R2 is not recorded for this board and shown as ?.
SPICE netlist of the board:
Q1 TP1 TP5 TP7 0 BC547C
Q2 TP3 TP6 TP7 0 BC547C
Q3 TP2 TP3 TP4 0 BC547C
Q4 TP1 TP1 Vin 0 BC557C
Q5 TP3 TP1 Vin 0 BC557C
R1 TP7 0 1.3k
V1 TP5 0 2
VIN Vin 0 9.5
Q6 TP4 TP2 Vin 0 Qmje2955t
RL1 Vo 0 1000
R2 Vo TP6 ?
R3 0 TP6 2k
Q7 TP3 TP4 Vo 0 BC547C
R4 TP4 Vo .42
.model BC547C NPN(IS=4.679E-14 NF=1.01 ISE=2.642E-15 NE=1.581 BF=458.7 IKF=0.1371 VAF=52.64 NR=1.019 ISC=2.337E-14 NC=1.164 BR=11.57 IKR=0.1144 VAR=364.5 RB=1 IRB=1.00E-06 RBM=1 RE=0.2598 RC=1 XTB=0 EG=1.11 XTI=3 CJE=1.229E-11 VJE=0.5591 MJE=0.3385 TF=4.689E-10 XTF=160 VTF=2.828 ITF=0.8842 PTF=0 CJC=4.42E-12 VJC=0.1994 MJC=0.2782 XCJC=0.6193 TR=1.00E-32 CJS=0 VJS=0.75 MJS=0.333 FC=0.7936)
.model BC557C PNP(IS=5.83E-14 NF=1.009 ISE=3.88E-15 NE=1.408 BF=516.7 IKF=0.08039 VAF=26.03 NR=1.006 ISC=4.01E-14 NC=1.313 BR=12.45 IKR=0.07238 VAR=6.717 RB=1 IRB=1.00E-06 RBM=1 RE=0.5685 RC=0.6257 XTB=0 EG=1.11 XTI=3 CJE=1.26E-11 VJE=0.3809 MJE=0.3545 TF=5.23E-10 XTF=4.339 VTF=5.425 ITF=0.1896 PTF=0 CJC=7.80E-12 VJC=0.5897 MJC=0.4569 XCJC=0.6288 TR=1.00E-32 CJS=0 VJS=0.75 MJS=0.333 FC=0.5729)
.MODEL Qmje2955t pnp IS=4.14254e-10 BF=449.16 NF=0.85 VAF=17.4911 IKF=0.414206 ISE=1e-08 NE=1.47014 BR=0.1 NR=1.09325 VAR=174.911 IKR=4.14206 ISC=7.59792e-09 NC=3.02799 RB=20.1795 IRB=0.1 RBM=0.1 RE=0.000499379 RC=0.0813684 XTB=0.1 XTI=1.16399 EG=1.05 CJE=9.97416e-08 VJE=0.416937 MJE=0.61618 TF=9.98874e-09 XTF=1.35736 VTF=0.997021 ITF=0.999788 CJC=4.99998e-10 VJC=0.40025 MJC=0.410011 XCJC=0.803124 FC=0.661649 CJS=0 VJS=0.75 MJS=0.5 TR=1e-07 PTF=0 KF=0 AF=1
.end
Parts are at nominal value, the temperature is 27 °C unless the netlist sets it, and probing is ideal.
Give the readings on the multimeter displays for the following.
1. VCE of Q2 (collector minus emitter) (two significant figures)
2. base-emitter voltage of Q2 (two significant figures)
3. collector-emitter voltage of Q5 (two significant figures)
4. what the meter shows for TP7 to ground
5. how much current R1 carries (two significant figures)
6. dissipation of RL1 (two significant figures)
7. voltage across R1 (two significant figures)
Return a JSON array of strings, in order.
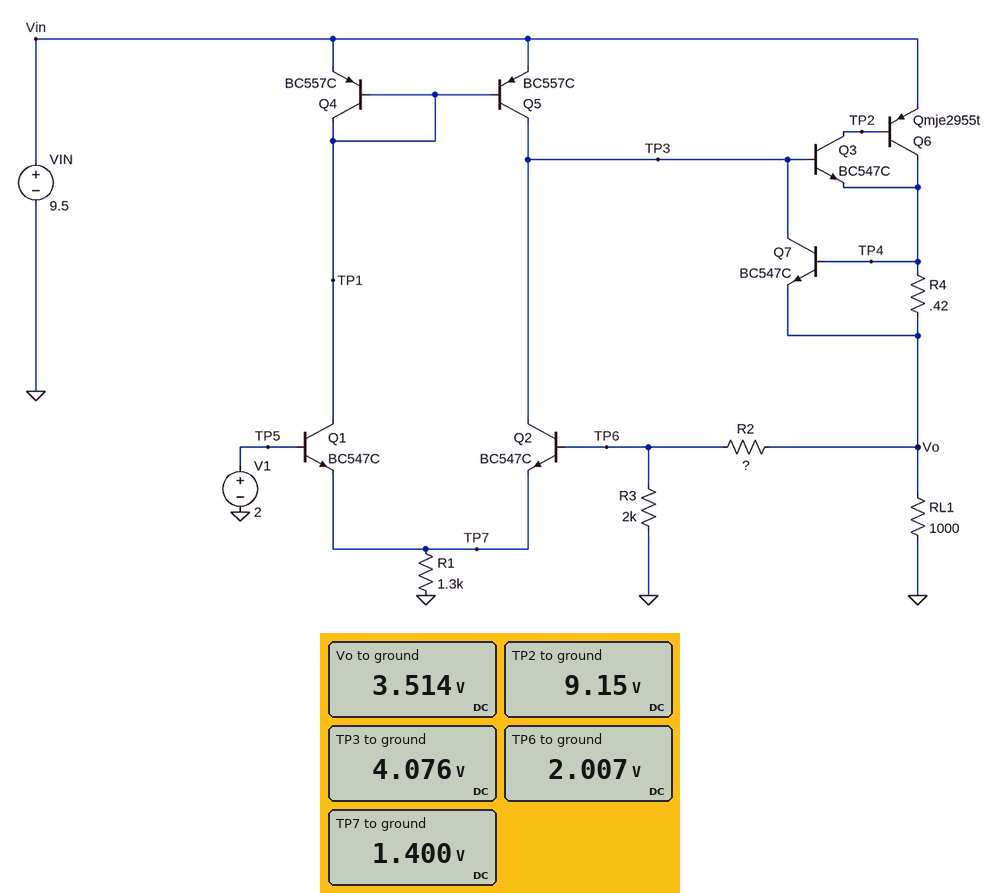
["2.7 V", "610 mV", "-5.4 V", "1.400 V", "1.1 mA", "12 mW", "1.4 V"]
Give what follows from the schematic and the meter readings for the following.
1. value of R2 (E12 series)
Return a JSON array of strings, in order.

["1.5 kΩ"]
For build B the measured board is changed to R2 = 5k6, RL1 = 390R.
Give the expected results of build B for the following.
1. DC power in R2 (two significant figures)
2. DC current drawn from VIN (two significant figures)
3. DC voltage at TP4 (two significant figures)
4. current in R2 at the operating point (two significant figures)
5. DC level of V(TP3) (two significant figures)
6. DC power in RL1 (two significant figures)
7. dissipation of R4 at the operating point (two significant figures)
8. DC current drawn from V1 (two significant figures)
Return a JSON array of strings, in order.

["5.6 mW", "22 mA", "7.6 V", "1.0 mA", "8.2 V", "150 mW", "180 µW", "1.0 µA"]
